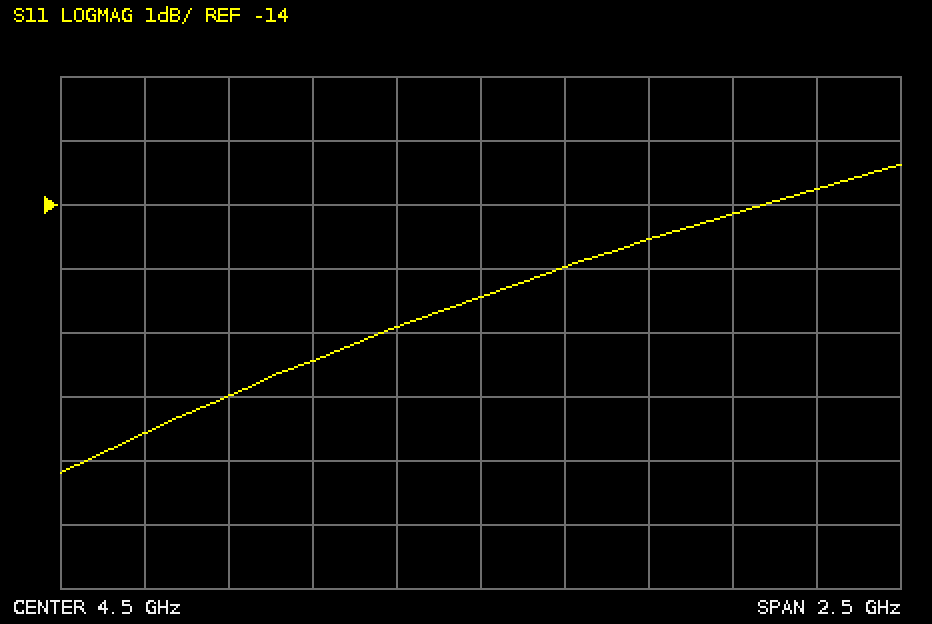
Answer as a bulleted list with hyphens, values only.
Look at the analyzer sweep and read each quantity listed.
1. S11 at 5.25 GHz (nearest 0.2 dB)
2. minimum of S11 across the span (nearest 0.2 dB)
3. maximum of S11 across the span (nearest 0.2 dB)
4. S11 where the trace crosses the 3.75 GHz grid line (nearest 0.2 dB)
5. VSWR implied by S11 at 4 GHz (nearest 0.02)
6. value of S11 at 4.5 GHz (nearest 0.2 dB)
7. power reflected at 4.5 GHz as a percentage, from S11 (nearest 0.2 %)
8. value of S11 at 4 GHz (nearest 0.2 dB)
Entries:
- -14.2 dB
- -18.2 dB
- -13.4 dB
- -17.0 dB
- 1.36
- -15.4 dB
- 2.8 %
- -16.4 dB
